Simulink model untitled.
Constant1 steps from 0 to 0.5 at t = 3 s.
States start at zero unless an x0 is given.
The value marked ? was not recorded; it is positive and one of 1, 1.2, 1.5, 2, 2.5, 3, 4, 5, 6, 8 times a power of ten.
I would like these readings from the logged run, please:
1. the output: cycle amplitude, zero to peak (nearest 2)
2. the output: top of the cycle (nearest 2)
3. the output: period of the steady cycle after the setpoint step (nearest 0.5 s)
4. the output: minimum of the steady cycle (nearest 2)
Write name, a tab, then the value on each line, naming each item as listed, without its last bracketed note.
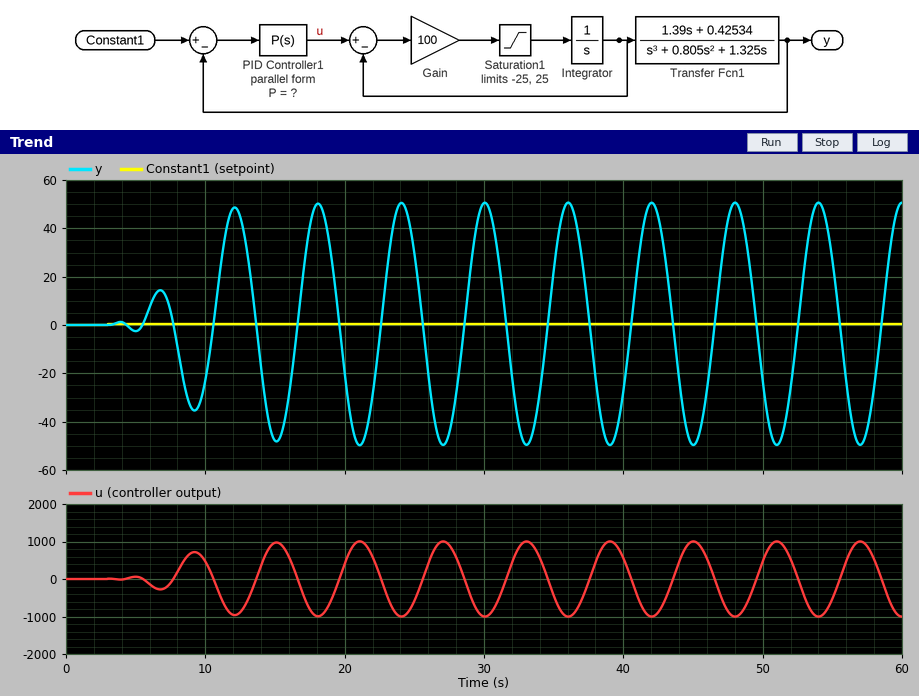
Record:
the output: cycle amplitude, zero to peak	50
the output: top of the cycle	50
the output: period of the steady cycle after the setpoint step	6.0 s
the output: minimum of the steady cycle	-50
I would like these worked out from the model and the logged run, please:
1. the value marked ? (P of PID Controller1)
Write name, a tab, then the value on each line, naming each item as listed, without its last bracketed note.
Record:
the value marked ?	20
